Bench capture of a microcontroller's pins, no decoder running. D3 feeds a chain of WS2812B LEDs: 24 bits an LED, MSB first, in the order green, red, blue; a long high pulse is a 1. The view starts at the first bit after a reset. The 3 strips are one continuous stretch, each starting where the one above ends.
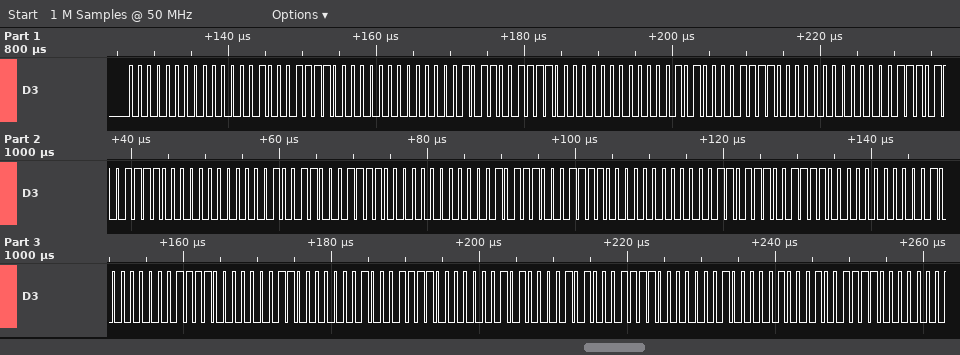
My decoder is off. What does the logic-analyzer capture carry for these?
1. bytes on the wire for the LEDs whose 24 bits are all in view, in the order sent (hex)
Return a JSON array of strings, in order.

["00 02 3C 00 0B 3C 00 14 3C 00 1D 3C 00 26 3C 00 2E 3C 00 37 3C 00 40 3C 06 02 3C 05 0A 3C 04 11 3C"]
